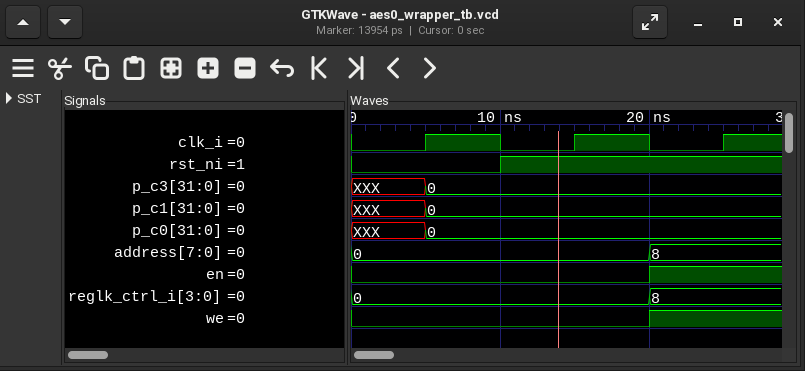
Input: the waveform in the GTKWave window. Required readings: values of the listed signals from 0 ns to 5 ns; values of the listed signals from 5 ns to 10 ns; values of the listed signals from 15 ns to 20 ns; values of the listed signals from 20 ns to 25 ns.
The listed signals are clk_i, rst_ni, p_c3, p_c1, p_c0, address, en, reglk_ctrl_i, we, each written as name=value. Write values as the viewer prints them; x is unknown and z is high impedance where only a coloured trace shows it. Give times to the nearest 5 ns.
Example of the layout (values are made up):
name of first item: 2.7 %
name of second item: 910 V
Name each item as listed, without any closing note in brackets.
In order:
values of the listed signals from 0 ns to 5 ns: clk_i=0, rst_ni=0, p_c3=XXX, p_c1=XXX, p_c0=XXX, address=0, en=0, reglk_ctrl_i=0, we=0
values of the listed signals from 5 ns to 10 ns: clk_i=1, rst_ni=0, p_c3=0, p_c1=0, p_c0=0, address=0, en=0, reglk_ctrl_i=0, we=0
values of the listed signals from 15 ns to 20 ns: clk_i=1, rst_ni=1, p_c3=0, p_c1=0, p_c0=0, address=0, en=0, reglk_ctrl_i=0, we=0
values of the listed signals from 20 ns to 25 ns: clk_i=0, rst_ni=1, p_c3=0, p_c1=0, p_c0=0, address=8, en=1, reglk_ctrl_i=8, we=1
